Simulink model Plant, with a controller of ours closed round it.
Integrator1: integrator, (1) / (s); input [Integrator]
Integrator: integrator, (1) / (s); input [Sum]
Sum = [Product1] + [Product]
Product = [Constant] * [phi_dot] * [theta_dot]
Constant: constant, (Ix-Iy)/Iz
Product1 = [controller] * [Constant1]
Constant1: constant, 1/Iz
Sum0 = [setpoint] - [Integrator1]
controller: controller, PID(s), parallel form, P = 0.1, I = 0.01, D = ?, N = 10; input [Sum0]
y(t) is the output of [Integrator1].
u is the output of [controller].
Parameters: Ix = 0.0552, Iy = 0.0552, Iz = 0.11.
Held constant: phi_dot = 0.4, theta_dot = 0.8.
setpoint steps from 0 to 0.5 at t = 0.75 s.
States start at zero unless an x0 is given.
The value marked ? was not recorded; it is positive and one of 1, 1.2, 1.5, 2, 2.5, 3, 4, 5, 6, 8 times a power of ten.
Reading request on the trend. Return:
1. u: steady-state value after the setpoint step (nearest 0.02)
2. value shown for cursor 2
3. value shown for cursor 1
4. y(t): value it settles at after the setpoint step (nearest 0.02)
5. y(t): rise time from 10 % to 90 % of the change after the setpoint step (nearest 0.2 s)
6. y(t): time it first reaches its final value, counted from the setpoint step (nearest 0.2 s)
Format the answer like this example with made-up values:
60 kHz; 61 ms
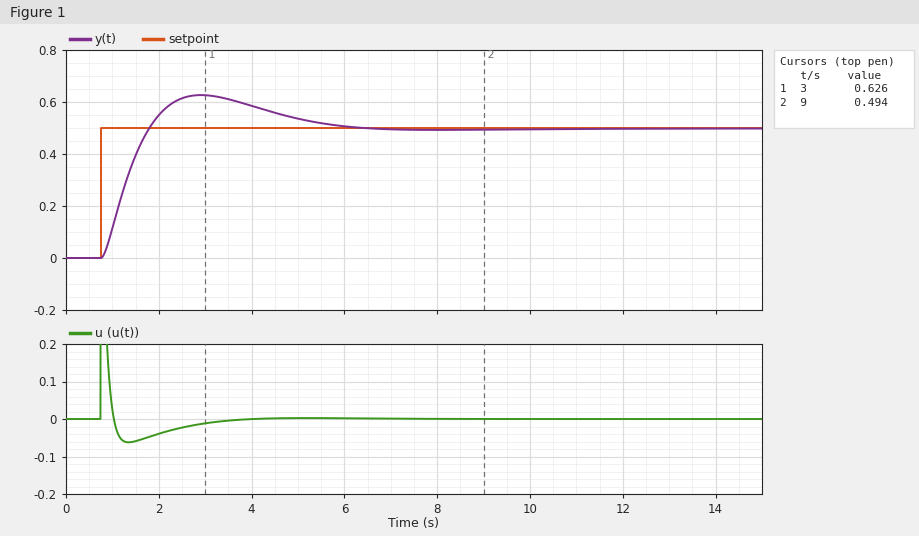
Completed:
0.00; 0.494; 0.626; 0.50; 0.8 s; 1.0 s
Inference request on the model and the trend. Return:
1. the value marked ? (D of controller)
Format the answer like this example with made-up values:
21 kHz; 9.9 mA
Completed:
0.15
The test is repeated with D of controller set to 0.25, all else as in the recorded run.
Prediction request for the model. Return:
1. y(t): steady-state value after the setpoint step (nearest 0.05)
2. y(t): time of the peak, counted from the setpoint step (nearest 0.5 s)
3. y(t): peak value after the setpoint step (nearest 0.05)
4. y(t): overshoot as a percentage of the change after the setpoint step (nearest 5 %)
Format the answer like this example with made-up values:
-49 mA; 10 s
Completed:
0.50; 1.5 s; 0.55; 15 %
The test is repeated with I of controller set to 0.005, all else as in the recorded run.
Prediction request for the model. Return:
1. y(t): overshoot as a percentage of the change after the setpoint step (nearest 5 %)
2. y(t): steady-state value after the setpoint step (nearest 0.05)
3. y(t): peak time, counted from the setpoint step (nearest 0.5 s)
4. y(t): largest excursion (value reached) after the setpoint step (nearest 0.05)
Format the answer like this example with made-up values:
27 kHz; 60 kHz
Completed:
25 %; 0.50; 2.0 s; 0.60
